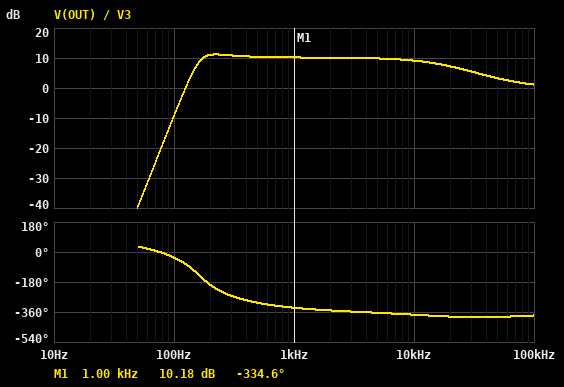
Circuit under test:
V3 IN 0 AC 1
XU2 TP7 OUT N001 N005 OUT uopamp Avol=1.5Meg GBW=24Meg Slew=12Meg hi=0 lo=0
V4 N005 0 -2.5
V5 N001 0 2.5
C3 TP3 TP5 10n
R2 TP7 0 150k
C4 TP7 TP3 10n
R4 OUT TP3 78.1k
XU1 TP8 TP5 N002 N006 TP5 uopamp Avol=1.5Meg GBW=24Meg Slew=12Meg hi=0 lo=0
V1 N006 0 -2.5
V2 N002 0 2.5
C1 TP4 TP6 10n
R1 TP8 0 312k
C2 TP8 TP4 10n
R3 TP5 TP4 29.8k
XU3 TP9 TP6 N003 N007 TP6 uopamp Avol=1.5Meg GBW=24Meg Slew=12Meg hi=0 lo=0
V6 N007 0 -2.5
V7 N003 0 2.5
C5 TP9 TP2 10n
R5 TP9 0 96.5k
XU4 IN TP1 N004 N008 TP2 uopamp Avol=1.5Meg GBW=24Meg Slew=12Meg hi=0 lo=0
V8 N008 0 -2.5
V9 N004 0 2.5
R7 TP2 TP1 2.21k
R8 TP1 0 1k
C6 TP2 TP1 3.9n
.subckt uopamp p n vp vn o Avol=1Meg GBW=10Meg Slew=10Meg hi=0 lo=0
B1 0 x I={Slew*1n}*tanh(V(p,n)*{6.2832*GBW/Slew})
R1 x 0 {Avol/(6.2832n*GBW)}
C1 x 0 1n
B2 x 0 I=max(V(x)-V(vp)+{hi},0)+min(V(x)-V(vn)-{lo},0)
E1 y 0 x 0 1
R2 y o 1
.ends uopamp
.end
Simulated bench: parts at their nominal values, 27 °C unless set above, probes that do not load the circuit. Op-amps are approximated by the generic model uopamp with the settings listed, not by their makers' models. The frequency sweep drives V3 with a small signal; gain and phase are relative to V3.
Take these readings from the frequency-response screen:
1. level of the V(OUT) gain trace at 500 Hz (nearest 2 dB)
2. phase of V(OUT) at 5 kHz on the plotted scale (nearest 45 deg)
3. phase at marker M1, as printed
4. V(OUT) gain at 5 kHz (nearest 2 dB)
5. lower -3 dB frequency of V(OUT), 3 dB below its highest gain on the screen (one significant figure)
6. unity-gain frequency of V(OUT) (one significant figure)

10 dB
-360 deg
-334.6 deg
10 dB
200 Hz
100 Hz
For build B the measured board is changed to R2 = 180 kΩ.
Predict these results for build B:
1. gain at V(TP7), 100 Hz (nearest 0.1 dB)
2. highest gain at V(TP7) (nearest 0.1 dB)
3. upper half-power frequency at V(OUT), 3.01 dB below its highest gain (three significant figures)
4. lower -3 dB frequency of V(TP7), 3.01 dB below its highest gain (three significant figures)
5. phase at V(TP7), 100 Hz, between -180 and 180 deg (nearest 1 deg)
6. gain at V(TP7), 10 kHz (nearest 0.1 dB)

-7.4 dB
12.0 dB
11.0 kHz
155 Hz
-38 deg
9.1 dB
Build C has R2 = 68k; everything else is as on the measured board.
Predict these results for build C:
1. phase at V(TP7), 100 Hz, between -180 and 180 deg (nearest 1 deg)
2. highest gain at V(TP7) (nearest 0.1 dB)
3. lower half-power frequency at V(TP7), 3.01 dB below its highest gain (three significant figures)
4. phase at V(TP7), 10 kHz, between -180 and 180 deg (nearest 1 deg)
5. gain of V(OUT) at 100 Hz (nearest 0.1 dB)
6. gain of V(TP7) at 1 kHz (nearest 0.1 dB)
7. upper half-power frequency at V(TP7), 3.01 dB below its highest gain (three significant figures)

-23 deg
10.0 dB
302 Hz
-15 deg
-17.2 dB
9.7 dB
21.3 kHz
